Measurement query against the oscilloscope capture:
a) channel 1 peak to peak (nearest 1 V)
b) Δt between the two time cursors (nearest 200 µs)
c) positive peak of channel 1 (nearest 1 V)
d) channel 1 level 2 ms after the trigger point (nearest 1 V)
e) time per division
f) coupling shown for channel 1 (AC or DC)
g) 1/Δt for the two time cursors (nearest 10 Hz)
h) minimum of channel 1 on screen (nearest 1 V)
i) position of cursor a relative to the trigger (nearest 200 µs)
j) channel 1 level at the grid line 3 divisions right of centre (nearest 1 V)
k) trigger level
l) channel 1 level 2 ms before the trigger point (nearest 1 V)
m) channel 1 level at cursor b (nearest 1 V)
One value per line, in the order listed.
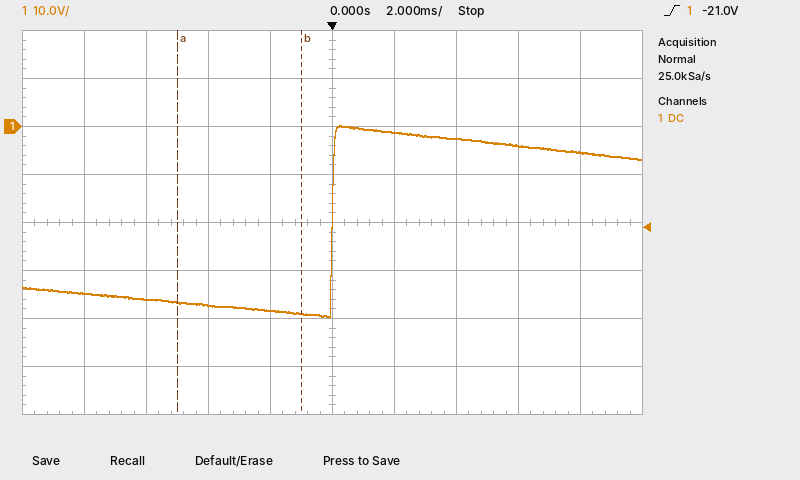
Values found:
40 V
4.0 ms
0 V
-1 V
2 ms
DC
250 Hz
-40 V
-5.0 ms
-4 V
-21.0 V
-38 V
-39 V
